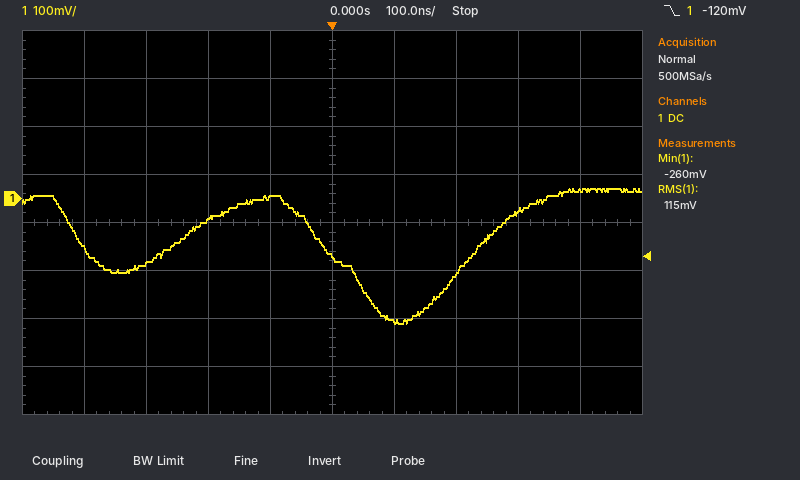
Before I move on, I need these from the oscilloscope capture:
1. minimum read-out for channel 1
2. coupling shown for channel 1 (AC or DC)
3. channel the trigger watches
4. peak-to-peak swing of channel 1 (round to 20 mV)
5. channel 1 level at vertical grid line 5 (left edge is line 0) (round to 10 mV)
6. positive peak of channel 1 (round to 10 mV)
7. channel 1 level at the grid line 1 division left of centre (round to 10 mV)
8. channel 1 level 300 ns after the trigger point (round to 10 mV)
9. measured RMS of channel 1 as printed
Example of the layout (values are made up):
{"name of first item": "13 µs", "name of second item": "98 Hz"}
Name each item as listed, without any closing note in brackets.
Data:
{"minimum read-out for channel 1": "-260 mV", "coupling shown for channel 1": "DC", "channel the trigger watches": "channel 1", "peak-to-peak swing of channel 1": "280 mV", "channel 1 level at vertical grid line 5 (left edge is line 0)": "-120 mV", "positive peak of channel 1": "20 mV", "channel 1 level at the grid line 1 division left of centre": "0 mV", "channel 1 level 300 ns after the trigger point": "-30 mV", "measured RMS of channel 1 as printed": "115 mV"}
